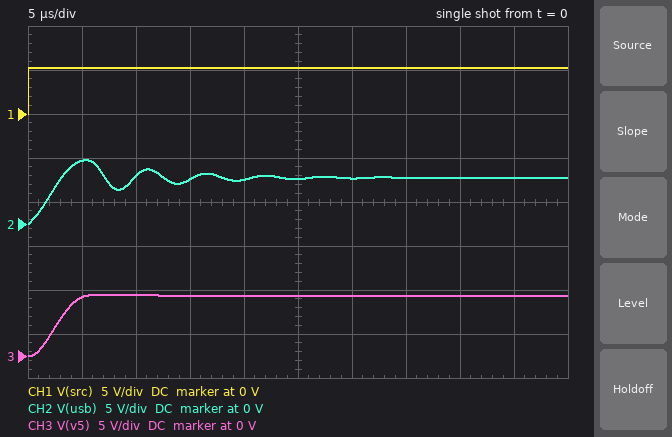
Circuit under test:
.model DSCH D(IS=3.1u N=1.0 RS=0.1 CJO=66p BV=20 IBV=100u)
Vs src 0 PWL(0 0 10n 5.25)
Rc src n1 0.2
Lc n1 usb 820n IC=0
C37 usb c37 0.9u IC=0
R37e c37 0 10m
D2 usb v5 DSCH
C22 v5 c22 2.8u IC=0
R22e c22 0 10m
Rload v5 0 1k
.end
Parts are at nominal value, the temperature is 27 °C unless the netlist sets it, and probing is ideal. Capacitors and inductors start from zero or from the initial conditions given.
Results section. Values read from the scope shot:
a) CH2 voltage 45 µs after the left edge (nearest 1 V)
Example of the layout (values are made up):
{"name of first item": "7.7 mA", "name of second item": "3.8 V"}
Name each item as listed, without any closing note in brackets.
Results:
{"CH2 voltage 45 µs after the left edge": "5 V"}
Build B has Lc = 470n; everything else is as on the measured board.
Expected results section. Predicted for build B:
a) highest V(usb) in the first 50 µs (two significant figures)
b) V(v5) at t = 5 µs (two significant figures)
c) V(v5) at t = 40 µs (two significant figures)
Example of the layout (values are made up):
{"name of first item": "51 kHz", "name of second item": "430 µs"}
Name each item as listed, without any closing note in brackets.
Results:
{"highest V(usb) in the first 50 µs": "6.7 V", "V(v5) at t = 5 µs": "6.3 V", "V(v5) at t = 40 µs": "6.2 V"}
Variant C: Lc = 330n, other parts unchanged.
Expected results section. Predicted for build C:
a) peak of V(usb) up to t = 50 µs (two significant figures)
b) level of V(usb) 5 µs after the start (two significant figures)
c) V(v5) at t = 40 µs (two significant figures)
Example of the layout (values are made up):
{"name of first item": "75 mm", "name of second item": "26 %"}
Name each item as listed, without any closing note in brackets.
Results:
{"peak of V(usb) up to t = 50 µs": "6.3 V", "level of V(usb) 5 µs after the start": "5.0 V", "V(v5) at t = 40 µs": "5.9 V"}
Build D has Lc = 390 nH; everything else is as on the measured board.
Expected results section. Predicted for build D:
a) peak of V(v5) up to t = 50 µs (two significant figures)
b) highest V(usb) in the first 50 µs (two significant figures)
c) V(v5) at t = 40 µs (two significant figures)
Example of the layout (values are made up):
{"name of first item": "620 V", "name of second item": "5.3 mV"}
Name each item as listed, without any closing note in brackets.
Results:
{"peak of V(v5) up to t = 50 µs": "6.1 V", "highest V(usb) in the first 50 µs": "6.5 V", "V(v5) at t = 40 µs": "6.0 V"}
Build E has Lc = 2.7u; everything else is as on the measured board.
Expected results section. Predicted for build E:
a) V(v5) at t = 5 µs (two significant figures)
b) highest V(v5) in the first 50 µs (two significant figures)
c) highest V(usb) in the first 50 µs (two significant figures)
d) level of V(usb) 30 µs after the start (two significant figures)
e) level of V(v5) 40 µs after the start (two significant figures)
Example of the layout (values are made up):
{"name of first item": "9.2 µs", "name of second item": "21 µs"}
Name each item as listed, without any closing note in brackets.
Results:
{"V(v5) at t = 5 µs": "4.2 V", "highest V(v5) in the first 50 µs": "8.0 V", "highest V(usb) in the first 50 µs": "8.3 V", "level of V(usb) 30 µs after the start": "6.6 V", "level of V(v5) 40 µs after the start": "7.9 V"}
